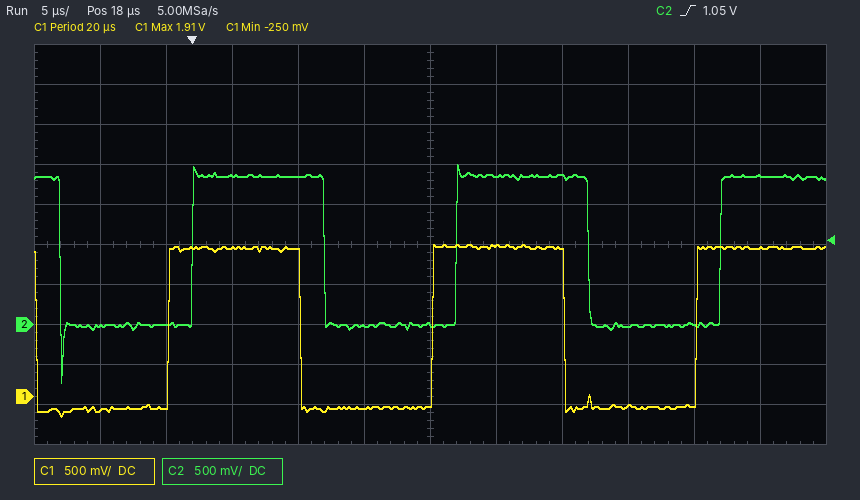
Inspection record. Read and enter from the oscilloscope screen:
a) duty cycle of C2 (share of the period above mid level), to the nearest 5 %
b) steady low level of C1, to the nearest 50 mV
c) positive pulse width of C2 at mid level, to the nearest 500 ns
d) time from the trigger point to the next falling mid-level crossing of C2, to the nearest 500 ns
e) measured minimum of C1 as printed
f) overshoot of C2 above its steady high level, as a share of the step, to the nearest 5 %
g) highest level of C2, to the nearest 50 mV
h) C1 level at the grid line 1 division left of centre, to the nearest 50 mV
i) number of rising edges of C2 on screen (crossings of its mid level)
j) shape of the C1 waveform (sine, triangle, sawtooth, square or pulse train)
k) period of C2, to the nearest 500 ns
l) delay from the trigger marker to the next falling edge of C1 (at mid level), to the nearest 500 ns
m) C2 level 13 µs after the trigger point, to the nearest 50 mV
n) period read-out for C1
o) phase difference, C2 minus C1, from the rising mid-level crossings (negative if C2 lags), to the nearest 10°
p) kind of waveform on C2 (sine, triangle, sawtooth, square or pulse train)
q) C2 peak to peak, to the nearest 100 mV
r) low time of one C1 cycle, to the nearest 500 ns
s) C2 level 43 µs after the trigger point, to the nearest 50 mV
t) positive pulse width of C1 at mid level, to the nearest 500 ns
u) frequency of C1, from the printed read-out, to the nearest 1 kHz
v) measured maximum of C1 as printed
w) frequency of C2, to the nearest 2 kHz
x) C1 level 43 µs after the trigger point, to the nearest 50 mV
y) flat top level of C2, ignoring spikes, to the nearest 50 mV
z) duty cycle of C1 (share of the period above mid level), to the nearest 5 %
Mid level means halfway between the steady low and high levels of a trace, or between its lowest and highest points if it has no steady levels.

50 %
-150 mV
10.0 µs
10.0 µs
-250 mV
10 %
2.00 V
-150 mV
3
square
20.0 µs
8.0 µs
0 mV
20 µs
-30°
square
2.70 V
10.0 µs
1.85 V
10.0 µs
50 kHz
1.91 V
50 kHz
1.85 V
1.85 V
50 %
